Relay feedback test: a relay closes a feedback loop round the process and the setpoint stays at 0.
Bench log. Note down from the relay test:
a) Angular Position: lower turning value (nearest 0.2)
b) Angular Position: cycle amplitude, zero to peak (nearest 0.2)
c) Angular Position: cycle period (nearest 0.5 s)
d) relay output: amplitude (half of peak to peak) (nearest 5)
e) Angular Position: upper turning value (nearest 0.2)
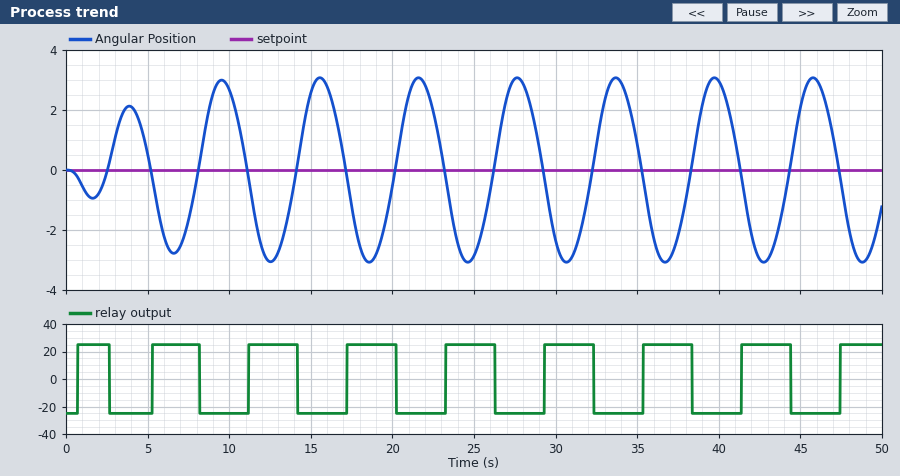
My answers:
-3.0
3.0
6.0 s
25
3.0
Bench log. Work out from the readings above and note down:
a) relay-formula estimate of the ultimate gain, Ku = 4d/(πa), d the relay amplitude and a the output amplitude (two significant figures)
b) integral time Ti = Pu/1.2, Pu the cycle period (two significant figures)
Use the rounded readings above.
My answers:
11
5.0 s
